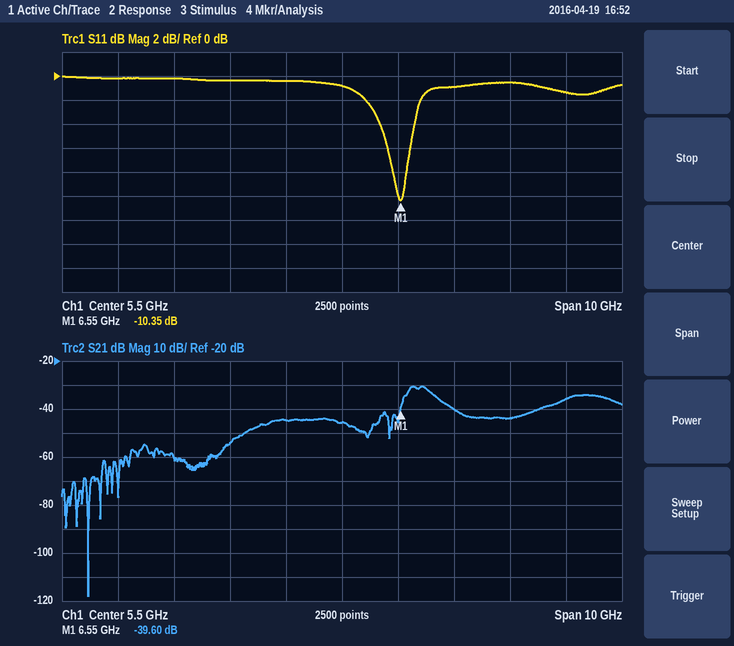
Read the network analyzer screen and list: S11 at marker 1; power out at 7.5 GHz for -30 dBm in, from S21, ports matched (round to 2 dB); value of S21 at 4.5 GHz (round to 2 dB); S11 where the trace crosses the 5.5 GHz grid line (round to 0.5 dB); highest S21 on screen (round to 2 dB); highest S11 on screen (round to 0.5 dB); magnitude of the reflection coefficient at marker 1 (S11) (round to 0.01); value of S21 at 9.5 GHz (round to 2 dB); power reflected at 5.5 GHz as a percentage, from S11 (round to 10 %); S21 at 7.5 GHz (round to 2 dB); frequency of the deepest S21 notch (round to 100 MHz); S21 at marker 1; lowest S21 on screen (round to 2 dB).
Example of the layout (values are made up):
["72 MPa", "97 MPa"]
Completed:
["-10.35 dB", "-70 dBm", "-44 dB", "-1.0 dB", "-30 dB", "0.0 dB", "0.30", "-36 dB", "80 %", "-40 dB", "1.0 GHz", "-39.60 dB", "-118 dB"]
